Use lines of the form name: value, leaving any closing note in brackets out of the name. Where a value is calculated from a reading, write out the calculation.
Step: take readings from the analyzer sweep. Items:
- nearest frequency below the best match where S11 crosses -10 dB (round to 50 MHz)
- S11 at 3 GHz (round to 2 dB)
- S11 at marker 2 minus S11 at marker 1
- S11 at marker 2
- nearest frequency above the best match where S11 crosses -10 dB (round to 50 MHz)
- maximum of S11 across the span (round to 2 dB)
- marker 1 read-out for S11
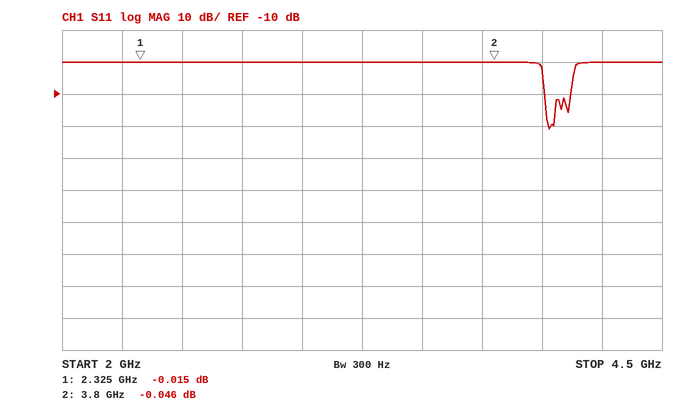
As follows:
nearest frequency below the best match where S11 crosses -10 dB: 4.00 GHz
S11 at 3 GHz: 0 dB
S11 at marker 2 minus S11 at marker 1: -0.046 − (-0.015) = -0.031 dB
S11 at marker 2: -0.046 dB
nearest frequency above the best match where S11 crosses -10 dB: 4.10 GHz
maximum of S11 across the span: 0 dB
marker 1 read-out for S11: -0.015 dB
